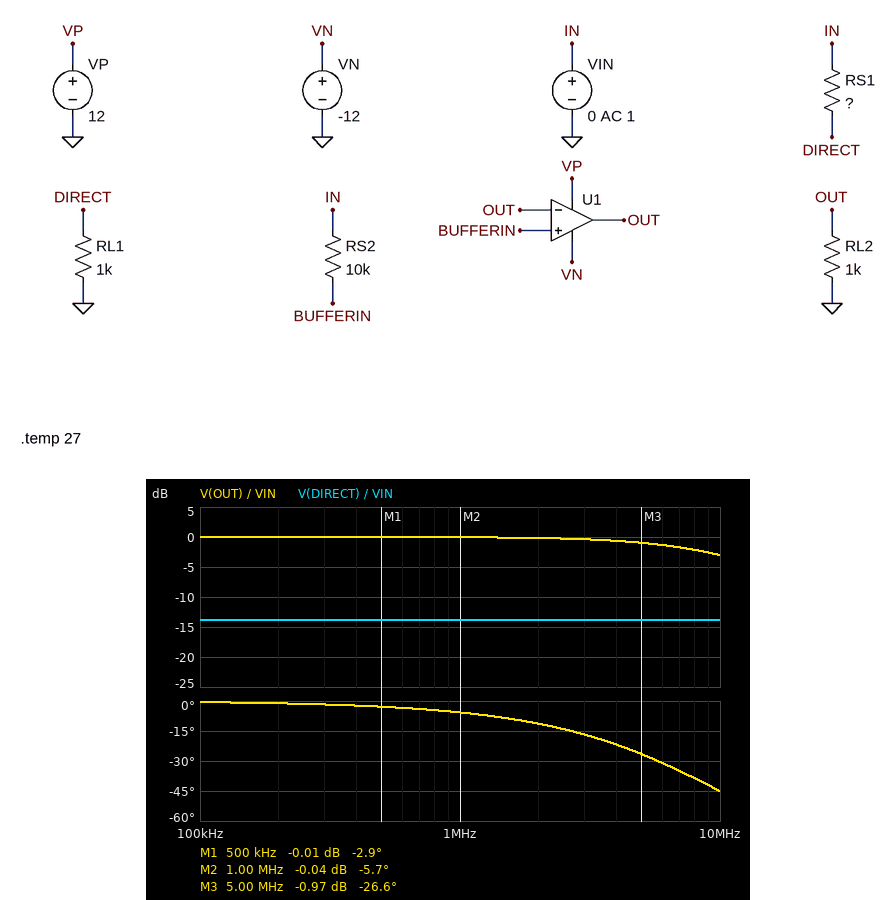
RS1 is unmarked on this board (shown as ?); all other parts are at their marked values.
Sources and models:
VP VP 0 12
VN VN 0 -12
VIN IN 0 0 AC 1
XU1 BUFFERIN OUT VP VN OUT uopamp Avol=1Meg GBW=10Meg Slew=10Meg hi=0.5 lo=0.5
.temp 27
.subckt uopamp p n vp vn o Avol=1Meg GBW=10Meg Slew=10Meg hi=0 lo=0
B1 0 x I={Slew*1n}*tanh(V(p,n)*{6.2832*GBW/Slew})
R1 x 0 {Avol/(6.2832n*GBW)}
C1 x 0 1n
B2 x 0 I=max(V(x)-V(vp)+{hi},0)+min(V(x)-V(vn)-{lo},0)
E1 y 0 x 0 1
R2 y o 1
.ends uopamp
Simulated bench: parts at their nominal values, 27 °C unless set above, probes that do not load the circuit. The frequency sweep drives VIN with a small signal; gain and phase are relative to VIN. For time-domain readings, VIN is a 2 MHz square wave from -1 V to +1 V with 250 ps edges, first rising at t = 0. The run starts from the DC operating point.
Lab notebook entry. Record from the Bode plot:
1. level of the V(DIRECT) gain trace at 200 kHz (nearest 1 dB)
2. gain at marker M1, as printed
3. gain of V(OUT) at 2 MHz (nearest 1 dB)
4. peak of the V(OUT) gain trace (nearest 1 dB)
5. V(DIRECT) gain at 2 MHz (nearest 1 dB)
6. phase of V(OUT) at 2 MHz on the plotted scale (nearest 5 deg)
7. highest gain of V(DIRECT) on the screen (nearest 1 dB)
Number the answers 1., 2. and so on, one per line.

1. -14 dB
2. -0.01 dB
3. 0 dB
4. 0 dB
5. -14 dB
6. -10 deg
7. -14 dB
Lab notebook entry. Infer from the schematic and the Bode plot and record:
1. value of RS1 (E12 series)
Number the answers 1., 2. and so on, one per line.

1. 3.9 kΩ
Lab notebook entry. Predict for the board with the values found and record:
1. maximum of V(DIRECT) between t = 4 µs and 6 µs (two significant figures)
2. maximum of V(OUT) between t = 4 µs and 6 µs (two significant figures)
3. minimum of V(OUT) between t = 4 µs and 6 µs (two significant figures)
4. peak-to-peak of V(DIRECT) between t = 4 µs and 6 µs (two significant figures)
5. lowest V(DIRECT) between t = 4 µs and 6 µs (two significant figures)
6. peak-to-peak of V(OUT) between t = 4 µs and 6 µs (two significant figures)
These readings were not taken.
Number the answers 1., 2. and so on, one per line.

1. 200 mV
2. 1.0 V
3. -1.0 V
4. 410 mV
5. -200 mV
6. 2.0 V
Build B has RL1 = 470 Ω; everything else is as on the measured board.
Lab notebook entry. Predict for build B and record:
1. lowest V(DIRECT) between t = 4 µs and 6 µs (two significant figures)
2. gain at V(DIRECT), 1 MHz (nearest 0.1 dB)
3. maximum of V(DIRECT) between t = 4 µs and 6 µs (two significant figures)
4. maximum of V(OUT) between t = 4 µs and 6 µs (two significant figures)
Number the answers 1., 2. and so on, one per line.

1. -110 mV
2. -19.4 dB
3. 110 mV
4. 1.0 V
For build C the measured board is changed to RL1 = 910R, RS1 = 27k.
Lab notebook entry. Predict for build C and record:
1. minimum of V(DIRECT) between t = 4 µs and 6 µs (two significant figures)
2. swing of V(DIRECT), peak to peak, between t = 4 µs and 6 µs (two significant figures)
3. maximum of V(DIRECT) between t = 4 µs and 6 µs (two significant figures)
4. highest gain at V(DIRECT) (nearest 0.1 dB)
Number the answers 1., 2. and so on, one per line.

1. -33 mV
2. 65 mV
3. 33 mV
4. -29.7 dB
